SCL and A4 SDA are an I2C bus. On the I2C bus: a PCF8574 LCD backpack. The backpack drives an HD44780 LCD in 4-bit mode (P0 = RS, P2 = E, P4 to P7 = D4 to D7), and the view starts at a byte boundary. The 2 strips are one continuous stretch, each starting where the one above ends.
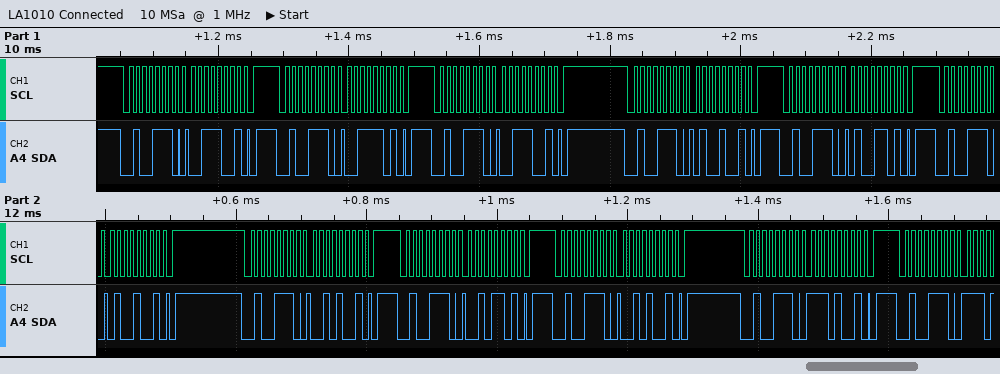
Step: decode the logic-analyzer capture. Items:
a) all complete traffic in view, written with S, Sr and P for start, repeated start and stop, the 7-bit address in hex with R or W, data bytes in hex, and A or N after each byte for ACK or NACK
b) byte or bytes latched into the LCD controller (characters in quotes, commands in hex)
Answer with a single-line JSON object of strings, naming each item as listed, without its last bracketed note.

{"all complete traffic in view, written with S, Sr and P for start, repeated start and stop, the 7-bit address in hex with R or W, data bytes in hex, and A or N after each byte for ACK or NACK": "S 27W A 39 A P S 27W A 3D A P S 27W A 39 A P S 27W A 49 A P S 27W A 4D A P S 27W A 49 A P S 27W A 29 A P S 27W A 2D A P S 27W A 29 A P S 27W A E9 A P S 27W A", "byte or bytes latched into the LCD controller": "'4'"}
